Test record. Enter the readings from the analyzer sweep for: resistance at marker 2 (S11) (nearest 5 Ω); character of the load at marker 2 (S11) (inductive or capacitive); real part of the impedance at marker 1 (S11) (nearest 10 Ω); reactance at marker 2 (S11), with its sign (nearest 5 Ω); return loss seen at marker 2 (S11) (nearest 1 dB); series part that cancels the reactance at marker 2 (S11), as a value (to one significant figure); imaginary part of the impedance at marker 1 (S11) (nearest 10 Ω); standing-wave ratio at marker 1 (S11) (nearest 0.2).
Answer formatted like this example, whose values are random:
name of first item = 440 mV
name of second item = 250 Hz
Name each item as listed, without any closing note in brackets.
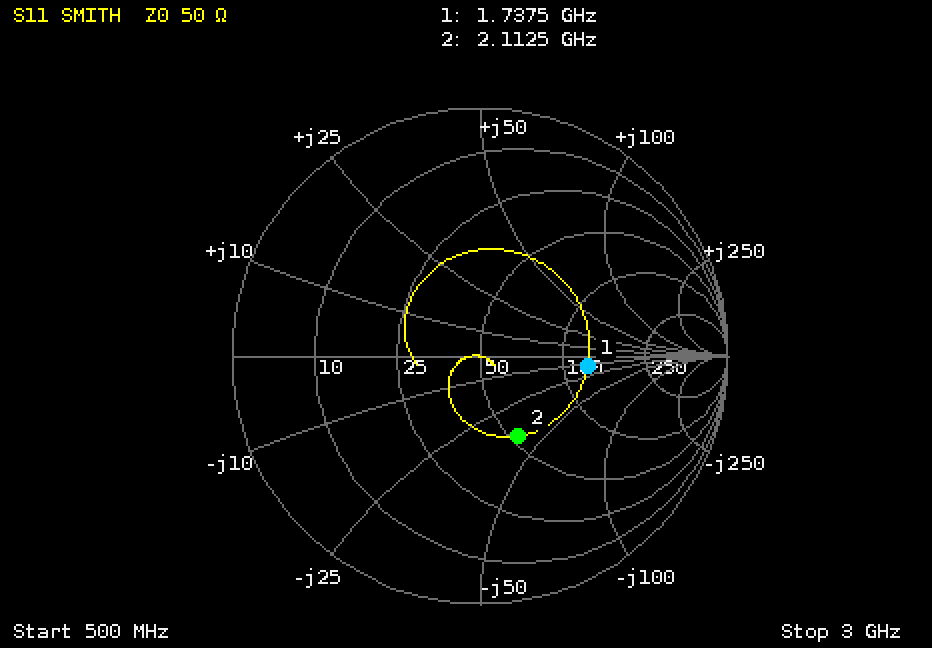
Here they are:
resistance at marker 2 (S11) = 55 Ω
character of the load at marker 2 (S11) = capacitive
real part of the impedance at marker 1 (S11) = 130 Ω
reactance at marker 2 (S11), with its sign = -40 Ω
return loss seen at marker 2 (S11) = 9 dB
series part that cancels the reactance at marker 2 (S11), as a value = 3 nH
imaginary part of the impedance at marker 1 (S11) = -10 Ω
standing-wave ratio at marker 1 (S11) = 2.6
